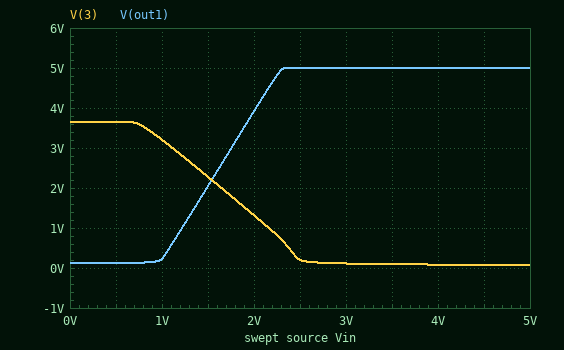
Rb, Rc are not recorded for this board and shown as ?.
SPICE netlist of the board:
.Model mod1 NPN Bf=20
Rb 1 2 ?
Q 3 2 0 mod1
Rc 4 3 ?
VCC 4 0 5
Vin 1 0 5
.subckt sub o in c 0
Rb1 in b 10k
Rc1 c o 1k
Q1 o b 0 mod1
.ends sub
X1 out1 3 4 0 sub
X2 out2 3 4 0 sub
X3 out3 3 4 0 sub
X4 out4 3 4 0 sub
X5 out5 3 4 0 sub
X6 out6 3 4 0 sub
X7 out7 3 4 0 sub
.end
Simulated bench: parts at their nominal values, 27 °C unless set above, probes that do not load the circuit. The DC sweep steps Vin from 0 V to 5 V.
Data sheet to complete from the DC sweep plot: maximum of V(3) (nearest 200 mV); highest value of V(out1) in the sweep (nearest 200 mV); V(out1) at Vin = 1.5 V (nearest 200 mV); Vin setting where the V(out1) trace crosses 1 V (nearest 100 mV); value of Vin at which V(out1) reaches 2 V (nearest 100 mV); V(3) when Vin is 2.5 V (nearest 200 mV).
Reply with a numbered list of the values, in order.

1. 3.6 V
2. 5.0 V
3. 2.0 V
4. 1.2 V
5. 1.5 V
6. 200 mV
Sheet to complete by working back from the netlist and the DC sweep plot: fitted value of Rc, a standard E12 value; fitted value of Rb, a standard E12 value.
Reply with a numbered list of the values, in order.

1. 680 Ω
2. 4.7 kΩ
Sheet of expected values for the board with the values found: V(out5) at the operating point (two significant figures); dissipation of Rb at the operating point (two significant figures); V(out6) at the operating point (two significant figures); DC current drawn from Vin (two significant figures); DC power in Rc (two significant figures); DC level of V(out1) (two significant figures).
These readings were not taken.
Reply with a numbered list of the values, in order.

1. 5.0 V
2. 3.7 mW
3. 5.0 V
4. 890 µA
5. 36 mW
6. 5.0 V
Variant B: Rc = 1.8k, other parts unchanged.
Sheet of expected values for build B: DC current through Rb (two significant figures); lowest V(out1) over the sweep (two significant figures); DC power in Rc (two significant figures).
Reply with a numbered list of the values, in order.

1. 890 µA
2. 1.3 V
3. 14 mW
